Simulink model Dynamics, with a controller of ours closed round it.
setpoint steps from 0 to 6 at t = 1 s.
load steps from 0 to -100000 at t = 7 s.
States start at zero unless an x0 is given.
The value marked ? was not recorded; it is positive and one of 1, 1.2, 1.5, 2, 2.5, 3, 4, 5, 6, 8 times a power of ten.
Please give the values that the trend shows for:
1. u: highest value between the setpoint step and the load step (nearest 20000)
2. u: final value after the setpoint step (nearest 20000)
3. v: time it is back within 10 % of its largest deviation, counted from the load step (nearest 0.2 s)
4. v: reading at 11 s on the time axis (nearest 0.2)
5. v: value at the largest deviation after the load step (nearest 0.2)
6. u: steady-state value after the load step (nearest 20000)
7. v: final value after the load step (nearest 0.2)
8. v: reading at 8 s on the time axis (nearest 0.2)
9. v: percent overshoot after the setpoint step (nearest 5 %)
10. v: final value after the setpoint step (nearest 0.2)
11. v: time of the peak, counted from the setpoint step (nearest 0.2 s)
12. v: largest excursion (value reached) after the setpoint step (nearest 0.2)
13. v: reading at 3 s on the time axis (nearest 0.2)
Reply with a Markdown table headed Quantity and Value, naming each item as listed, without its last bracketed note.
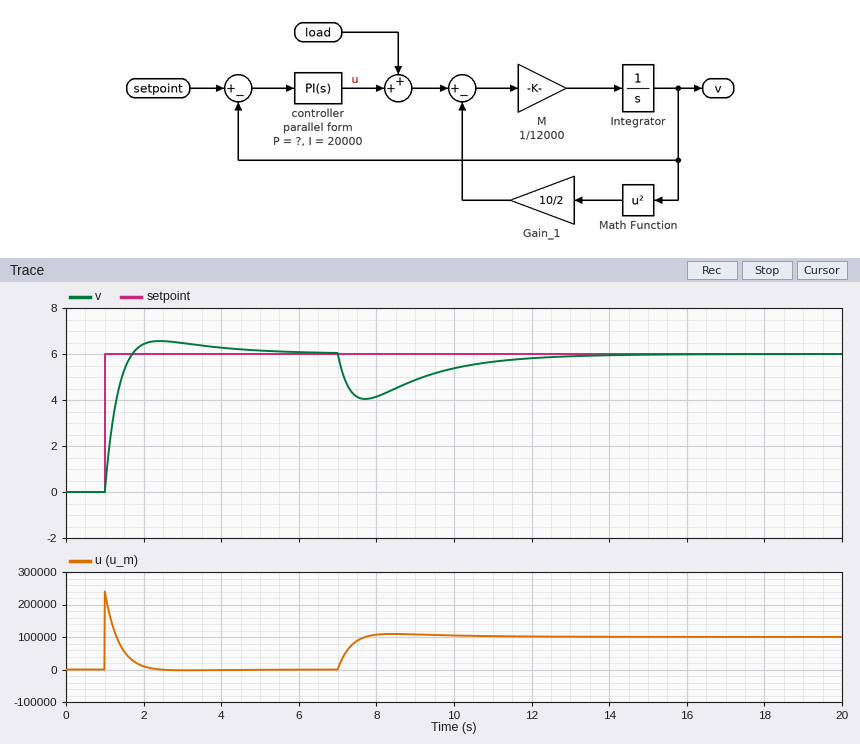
| Quantity | Value |
|---|---|
| u: highest value between the setpoint step and the load step | 240000 |
| u: final value after the setpoint step | 0 |
| v: time it is back within 10 % of its largest deviation, counted from the load step | 4.8 s |
| v: reading at 11 s on the time axis | 5.6 |
| v: value at the largest deviation after the load step | 4.0 |
| u: steady-state value after the load step | 100000 |
| v: final value after the load step | 6.0 |
| v: reading at 8 s on the time axis | 4.2 |
| v: percent overshoot after the setpoint step | 10 % |
| v: final value after the setpoint step | 6.0 |
| v: time of the peak, counted from the setpoint step | 1.4 s |
| v: largest excursion (value reached) after the setpoint step | 6.6 |
| v: reading at 3 s on the time axis | 6.4 |
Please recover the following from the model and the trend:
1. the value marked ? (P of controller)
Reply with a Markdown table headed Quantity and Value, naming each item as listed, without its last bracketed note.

| Quantity | Value |
|---|---|
| the value marked ? | 40000 |
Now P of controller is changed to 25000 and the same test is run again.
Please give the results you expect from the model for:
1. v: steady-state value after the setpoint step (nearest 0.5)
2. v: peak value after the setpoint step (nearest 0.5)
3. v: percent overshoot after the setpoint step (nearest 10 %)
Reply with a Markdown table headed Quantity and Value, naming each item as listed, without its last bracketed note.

| Quantity | Value |
|---|---|
| v: steady-state value after the setpoint step | 6.0 |
| v: peak value after the setpoint step | 7.0 |
| v: percent overshoot after the setpoint step | 20 % |
